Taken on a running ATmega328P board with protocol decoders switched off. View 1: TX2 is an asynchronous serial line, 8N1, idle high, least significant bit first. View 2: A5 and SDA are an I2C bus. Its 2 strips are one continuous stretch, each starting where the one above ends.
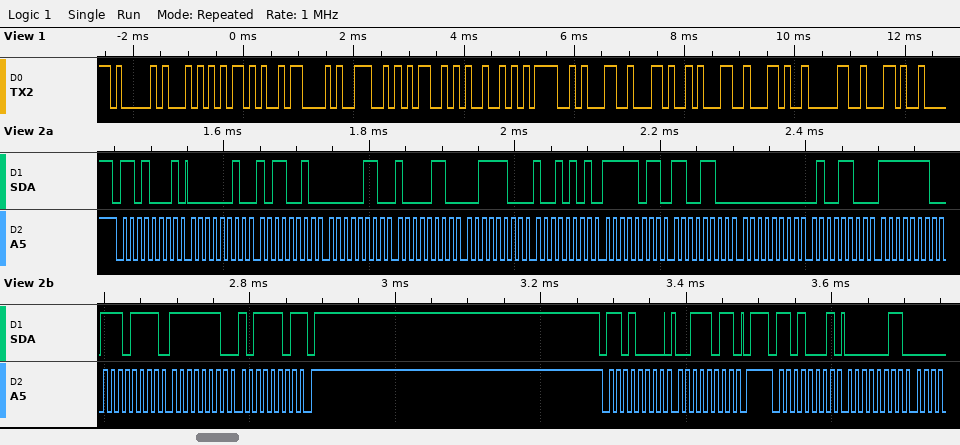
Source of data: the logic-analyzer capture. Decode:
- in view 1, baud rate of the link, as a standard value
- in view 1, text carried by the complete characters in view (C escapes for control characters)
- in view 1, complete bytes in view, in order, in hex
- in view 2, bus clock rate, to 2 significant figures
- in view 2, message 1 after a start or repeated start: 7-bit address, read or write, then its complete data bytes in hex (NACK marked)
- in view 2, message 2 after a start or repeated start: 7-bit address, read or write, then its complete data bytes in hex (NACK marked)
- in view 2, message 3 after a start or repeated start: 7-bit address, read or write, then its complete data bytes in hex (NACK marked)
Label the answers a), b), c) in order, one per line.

a) 9600 baud
b) "AT+CNMI=1,1,0,"
c) 41 54 2B 43 4E 4D 49 3D 31 2C 31 2C 30 2C
d) 100 kHz
e) 0x68 read: 02 B2 06 86 3C 95 FB CC 00 4C FE EF FE BD NACK
f) 0x68 write: 3B
g) 0x68 read: 03
